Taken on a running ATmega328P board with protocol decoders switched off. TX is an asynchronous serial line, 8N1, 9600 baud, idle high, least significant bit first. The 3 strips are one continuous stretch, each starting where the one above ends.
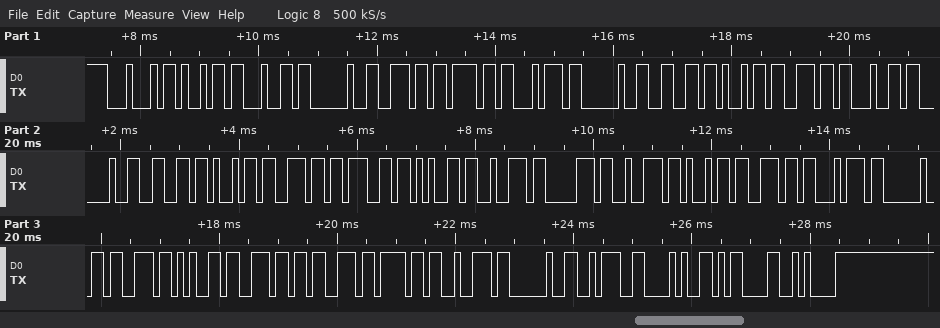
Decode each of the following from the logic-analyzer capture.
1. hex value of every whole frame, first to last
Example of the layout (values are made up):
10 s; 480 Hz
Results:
0x44 0x69 0x64 0x20 0x6E 0x6F 0x74 0x20 0x66 0x69 0x6E 0x64 0x20 0x66 0x69 0x6E 0x67 0x65 0x72 0x70 0x72 0x69 0x6E 0x74 0x20 0x73 0x65 0x6E 0x73 0x6F 0x72 0x20 0x3A 0x28 0x0D 0x0A
